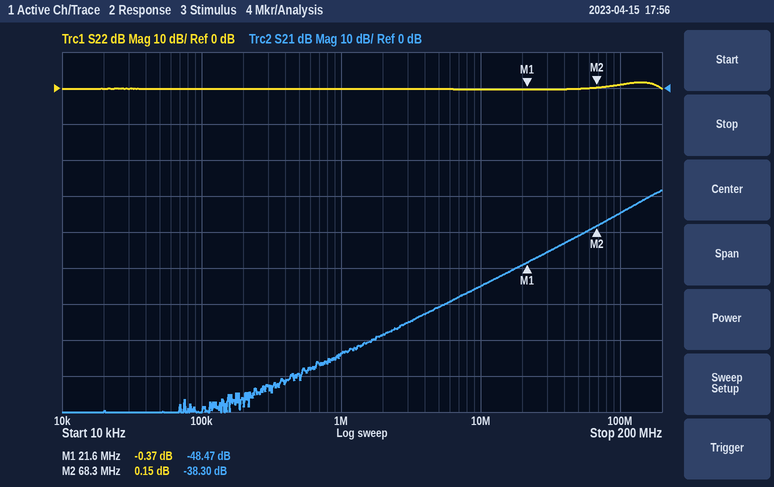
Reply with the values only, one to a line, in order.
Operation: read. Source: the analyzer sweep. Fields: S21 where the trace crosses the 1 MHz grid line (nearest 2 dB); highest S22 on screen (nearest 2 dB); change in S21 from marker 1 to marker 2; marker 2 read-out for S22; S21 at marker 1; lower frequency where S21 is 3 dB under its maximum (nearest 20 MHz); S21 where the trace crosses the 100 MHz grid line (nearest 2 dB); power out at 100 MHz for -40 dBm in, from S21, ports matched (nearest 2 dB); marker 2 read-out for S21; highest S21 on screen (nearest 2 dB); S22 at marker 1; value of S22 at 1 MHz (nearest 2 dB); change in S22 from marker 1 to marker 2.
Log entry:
-74 dB
2 dB
10.17 dB
0.15 dB
-48.47 dB
140 MHz
-34 dB
-74 dBm
-38.30 dB
-28 dB
-0.37 dB
0 dB
0.52 dB
